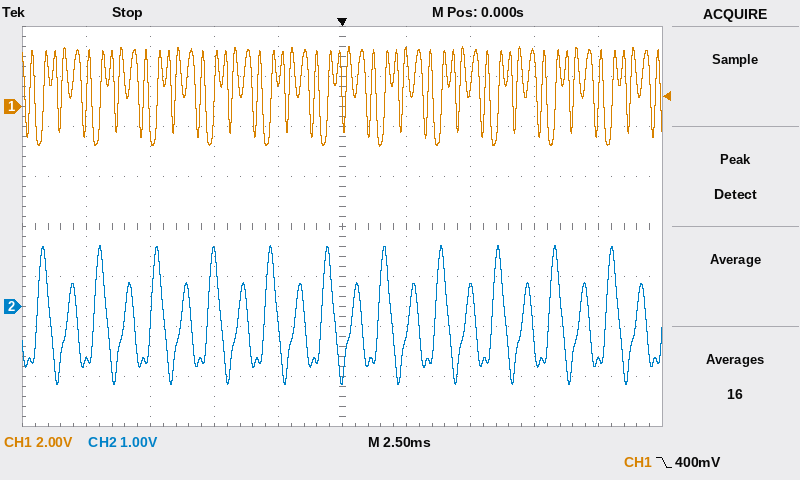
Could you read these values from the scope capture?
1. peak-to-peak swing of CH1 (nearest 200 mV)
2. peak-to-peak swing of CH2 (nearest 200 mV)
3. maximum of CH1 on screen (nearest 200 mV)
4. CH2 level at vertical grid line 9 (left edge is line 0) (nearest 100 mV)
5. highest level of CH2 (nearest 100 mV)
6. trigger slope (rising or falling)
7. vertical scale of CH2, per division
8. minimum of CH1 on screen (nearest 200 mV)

4.0 V
2.8 V
2.4 V
-1.1 V
1.2 V
falling
1 V
-1.6 V
